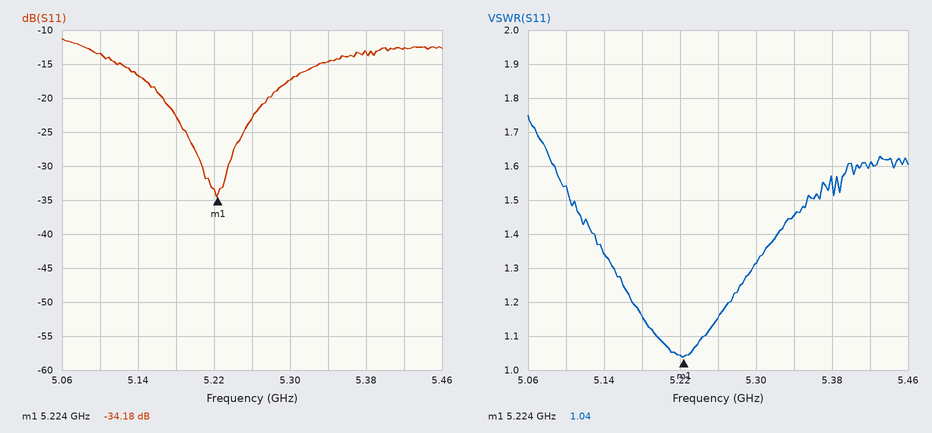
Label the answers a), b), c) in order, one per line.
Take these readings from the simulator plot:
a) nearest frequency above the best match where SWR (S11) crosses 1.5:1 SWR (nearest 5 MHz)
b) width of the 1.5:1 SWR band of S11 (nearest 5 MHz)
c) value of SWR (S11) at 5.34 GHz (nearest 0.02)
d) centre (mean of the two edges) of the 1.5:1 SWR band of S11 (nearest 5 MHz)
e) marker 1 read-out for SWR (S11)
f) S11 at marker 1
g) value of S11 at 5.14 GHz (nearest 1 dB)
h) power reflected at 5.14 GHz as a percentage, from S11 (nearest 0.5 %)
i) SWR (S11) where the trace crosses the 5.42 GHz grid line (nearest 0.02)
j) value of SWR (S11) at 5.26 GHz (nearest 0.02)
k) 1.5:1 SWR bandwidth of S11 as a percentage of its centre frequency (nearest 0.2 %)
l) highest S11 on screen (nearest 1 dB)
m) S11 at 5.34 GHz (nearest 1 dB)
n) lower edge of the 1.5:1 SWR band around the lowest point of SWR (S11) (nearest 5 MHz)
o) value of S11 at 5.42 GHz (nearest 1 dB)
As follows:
a) 5.355 GHz
b) 250 MHz
c) 1.46
d) 5.230 GHz
e) 1.04
f) -34.18 dB
g) -17 dB
h) 2.0 %
i) 1.60
j) 1.16
k) 4.8 %
l) -11 dB
m) -15 dB
n) 5.105 GHz
o) -13 dB
